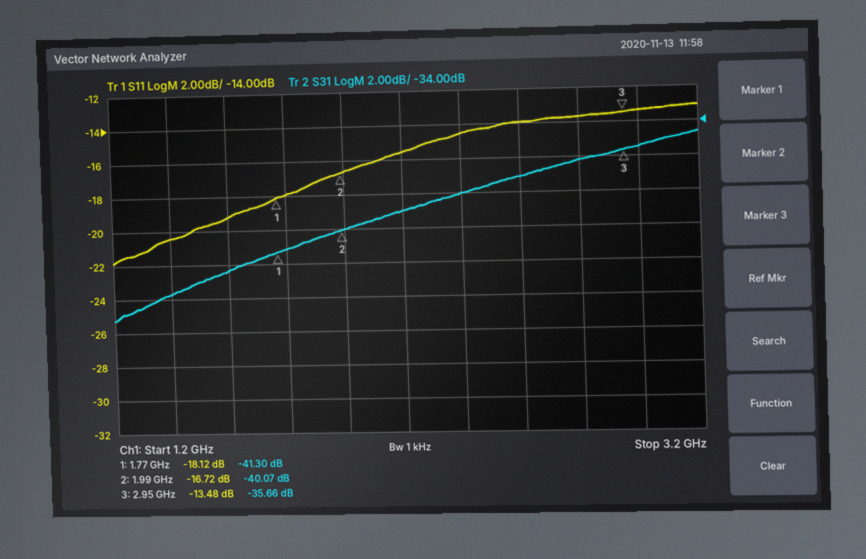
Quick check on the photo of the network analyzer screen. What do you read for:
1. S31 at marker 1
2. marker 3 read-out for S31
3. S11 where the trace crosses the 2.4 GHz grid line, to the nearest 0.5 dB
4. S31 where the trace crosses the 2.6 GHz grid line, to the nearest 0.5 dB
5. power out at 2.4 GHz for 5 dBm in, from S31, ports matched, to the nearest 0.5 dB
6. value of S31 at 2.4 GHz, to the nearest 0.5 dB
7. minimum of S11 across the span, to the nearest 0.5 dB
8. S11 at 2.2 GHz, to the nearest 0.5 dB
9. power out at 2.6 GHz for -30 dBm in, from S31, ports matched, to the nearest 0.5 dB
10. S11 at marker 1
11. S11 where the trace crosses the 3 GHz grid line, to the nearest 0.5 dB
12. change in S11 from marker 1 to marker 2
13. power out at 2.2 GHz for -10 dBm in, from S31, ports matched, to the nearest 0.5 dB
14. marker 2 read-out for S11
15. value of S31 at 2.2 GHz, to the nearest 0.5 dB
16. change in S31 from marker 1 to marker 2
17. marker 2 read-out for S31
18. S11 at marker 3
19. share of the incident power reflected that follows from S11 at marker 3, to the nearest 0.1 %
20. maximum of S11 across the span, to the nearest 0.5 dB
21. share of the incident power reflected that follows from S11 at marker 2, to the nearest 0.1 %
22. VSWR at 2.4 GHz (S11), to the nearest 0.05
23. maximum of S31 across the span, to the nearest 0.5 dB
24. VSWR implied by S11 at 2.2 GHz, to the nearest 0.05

-41.30 dB
-35.66 dB
-14.5 dB
-37.0 dB
-33.0 dBm
-38.0 dB
-22.0 dB
-15.5 dB
-67.0 dBm
-18.12 dB
-13.5 dB
1.40 dB
-49.0 dBm
-16.72 dB
-39.0 dB
1.23 dB
-40.07 dB
-13.48 dB
4.5 %
-13.0 dB
2.1 %
1.45
-34.5 dB
1.40
